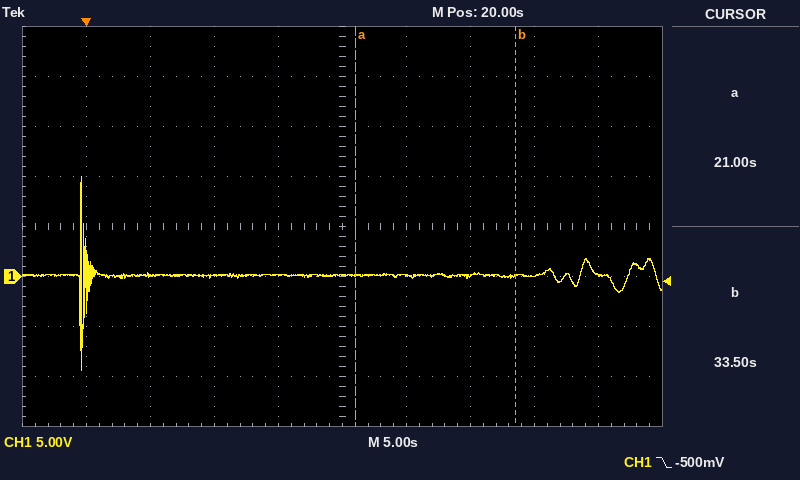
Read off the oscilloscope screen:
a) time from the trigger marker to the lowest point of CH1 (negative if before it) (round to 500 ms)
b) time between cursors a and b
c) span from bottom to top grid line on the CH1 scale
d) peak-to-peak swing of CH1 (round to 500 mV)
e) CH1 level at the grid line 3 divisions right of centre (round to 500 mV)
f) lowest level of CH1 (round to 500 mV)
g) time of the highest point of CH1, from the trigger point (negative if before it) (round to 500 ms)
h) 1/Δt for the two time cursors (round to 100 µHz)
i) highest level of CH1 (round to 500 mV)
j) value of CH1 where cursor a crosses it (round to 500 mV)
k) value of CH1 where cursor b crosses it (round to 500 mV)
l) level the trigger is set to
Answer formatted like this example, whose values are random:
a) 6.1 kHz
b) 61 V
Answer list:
a) -500 ms
b) 12.5 s
c) 40 V
d) 19.5 V
e) 0.0 V
f) -9.5 V
g) -500 ms
h) 80.0 mHz
i) 10.0 V
j) 0.0 V
k) 0.0 V
l) -500 mV
